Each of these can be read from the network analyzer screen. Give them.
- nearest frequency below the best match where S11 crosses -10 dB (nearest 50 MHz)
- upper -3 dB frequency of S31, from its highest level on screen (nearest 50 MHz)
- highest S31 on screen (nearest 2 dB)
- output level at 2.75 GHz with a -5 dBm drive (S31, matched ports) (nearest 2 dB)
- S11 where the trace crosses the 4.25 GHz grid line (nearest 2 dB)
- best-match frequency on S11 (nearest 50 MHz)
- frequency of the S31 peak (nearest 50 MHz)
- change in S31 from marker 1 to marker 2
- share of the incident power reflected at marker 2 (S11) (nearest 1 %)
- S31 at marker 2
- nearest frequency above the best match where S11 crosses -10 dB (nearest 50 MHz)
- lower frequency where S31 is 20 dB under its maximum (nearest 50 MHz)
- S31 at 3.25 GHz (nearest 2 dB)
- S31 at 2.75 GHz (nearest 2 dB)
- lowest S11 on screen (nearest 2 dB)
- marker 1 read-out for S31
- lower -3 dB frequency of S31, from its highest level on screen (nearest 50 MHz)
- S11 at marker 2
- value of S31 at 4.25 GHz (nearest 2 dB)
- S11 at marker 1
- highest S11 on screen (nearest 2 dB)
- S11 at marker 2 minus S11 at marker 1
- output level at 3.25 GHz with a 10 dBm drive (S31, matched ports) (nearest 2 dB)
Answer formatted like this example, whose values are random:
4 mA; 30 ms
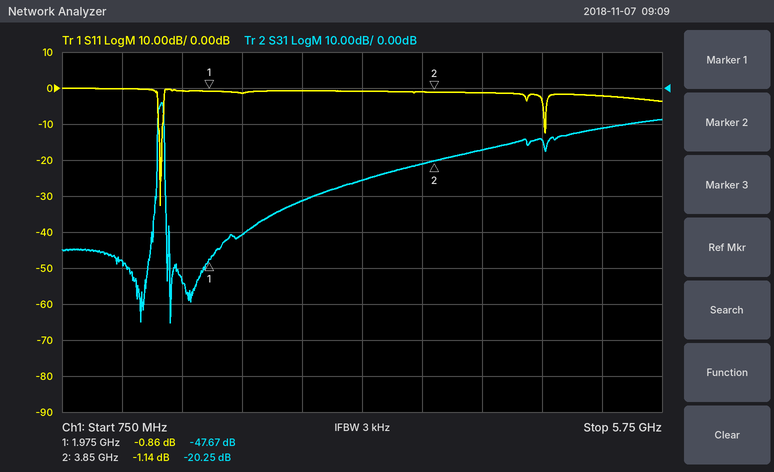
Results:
1.55 GHz; 1.60 GHz; -4 dB; -36 dBm; -2 dB; 1.55 GHz; 1.60 GHz; 27.42 dB; 77 %; -20.25 dB; 1.60 GHz; 1.55 GHz; -26 dB; -32 dB; -32 dB; -47.67 dB; 1.55 GHz; -1.14 dB; -18 dB; -0.86 dB; 0 dB; -0.28 dB; -16 dBm
